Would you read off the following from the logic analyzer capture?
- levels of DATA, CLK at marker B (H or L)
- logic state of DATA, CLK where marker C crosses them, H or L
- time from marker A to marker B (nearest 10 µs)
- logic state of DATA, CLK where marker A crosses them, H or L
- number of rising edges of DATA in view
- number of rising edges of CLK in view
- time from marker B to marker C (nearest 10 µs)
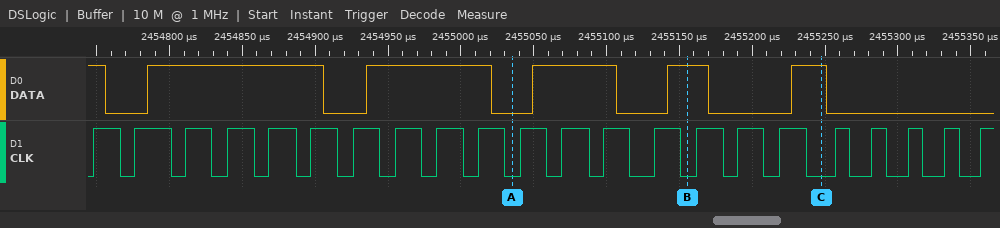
DATA=H, CLK=L
DATA=H, CLK=L
120 µs
DATA=L, CLK=L
5
22
90 µs
